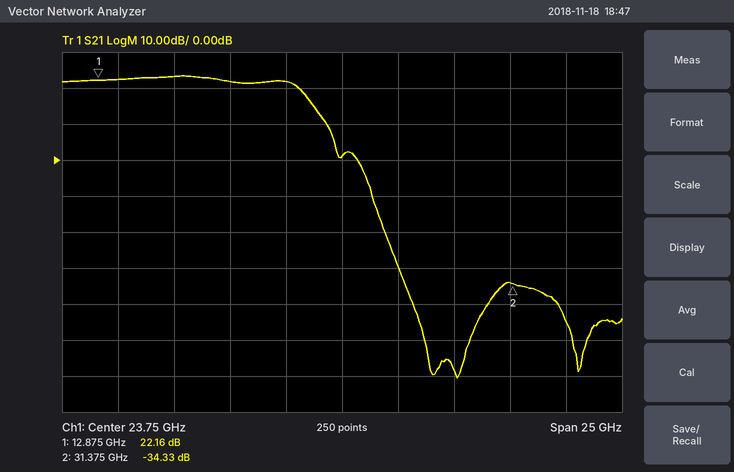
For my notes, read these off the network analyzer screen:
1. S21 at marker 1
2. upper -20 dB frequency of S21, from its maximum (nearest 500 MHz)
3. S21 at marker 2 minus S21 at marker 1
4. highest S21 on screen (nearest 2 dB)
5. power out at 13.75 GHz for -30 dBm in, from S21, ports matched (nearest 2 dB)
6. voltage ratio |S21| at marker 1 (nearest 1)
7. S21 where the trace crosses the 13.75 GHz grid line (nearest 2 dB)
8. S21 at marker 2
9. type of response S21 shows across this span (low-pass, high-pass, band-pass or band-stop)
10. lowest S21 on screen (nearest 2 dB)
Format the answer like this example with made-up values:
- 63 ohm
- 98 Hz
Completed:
- 22.16 dB
- 23.5 GHz
- -56.49 dB
- 24 dB
- -8 dBm
- 13
- 22 dB
- -34.33 dB
- low-pass
- -60 dB
